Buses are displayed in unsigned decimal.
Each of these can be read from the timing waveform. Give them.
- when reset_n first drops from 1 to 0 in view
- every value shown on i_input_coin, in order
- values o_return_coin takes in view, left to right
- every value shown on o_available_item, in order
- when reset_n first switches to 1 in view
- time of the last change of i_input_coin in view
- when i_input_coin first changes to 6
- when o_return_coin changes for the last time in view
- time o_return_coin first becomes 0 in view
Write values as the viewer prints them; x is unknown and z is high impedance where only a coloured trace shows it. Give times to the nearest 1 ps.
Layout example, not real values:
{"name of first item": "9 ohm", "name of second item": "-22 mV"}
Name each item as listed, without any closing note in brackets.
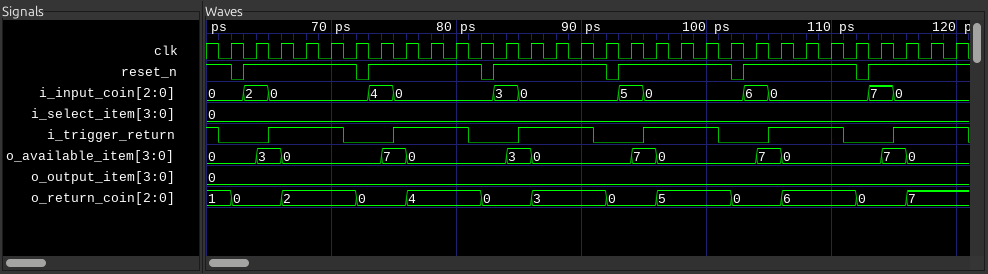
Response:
{"when reset_n first drops from 1 to 0 in view": "62 ps", "every value shown on i_input_coin, in order": "0, 2, 0, 4, 0, 3, 0, 5, 0, 6, 0, 7, 0", "values o_return_coin takes in view, left to right": "1, 0, 2, 0, 4, 0, 3, 0, 5, 0, 6, 0, 7", "every value shown on o_available_item, in order": "0, 3, 0, 7, 0, 3, 0, 7, 0, 7, 0, 7, 0", "when reset_n first switches to 1 in view": "63 ps", "time of the last change of i_input_coin in view": "115 ps", "when i_input_coin first changes to 6": "103 ps", "when o_return_coin changes for the last time in view": "116 ps", "time o_return_coin first becomes 0 in view": "62 ps"}
